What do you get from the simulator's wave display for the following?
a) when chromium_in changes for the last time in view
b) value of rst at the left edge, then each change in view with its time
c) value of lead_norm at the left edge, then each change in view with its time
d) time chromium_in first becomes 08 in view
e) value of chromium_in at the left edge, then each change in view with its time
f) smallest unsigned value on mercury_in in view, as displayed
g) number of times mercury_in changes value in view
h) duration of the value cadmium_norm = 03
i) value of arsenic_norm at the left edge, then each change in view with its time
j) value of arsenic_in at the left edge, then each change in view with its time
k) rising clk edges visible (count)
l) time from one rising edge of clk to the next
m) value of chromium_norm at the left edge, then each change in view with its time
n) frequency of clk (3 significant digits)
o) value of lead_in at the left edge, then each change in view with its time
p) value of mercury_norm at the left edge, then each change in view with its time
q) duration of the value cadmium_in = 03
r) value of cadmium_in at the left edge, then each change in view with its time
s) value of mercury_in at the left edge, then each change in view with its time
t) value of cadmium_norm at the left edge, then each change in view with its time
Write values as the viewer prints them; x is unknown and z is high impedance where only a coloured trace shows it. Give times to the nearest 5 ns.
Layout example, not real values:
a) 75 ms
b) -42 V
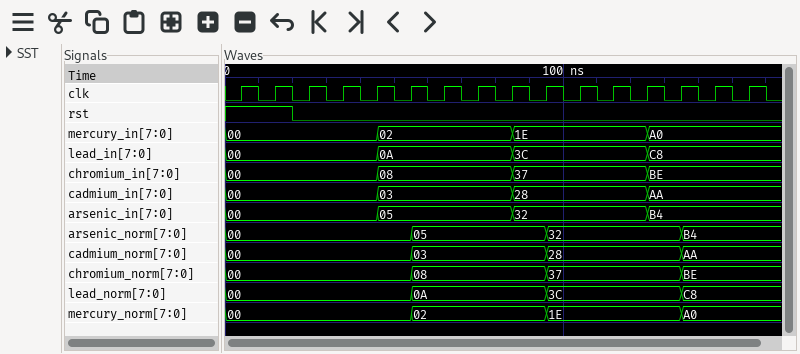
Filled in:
a) 125 ns
b) 1, 0 at 20 ns
c) 00, 0A at 55 ns, 3C at 95 ns, C8 at 135 ns
d) 45 ns
e) 00, 08 at 45 ns, 37 at 85 ns, BE at 125 ns
f) 00
g) 3
h) 40 ns
i) 00, 05 at 55 ns, 32 at 95 ns, B4 at 135 ns
j) 00, 05 at 45 ns, 32 at 85 ns, B4 at 125 ns
k) 16
l) 10 ns
m) 00, 08 at 55 ns, 37 at 95 ns, BE at 135 ns
n) 100 MHz
o) 00, 0A at 45 ns, 3C at 85 ns, C8 at 125 ns
p) 00, 02 at 55 ns, 1E at 95 ns, A0 at 135 ns
q) 40 ns
r) 00, 03 at 45 ns, 28 at 85 ns, AA at 125 ns
s) 00, 02 at 45 ns, 1E at 85 ns, A0 at 125 ns
t) 00, 03 at 55 ns, 28 at 95 ns, AA at 135 ns
